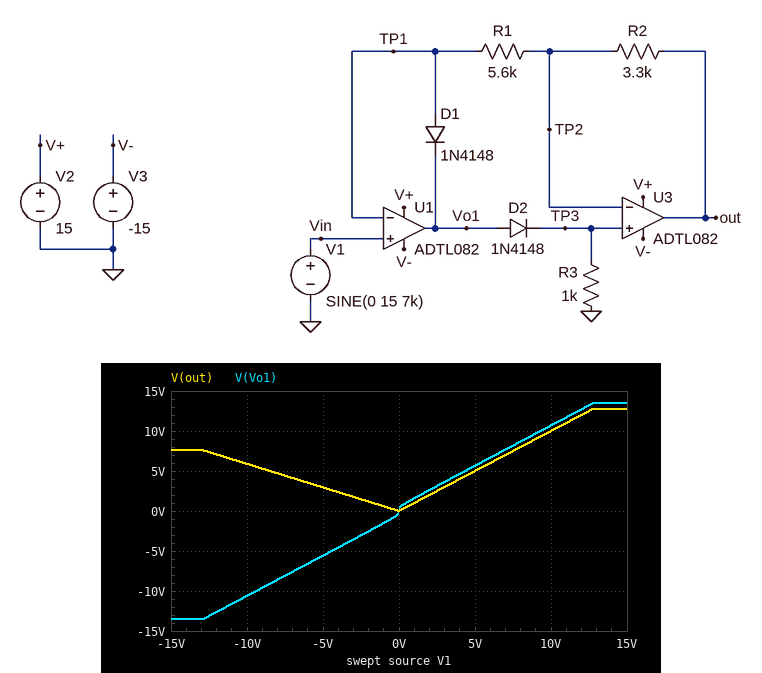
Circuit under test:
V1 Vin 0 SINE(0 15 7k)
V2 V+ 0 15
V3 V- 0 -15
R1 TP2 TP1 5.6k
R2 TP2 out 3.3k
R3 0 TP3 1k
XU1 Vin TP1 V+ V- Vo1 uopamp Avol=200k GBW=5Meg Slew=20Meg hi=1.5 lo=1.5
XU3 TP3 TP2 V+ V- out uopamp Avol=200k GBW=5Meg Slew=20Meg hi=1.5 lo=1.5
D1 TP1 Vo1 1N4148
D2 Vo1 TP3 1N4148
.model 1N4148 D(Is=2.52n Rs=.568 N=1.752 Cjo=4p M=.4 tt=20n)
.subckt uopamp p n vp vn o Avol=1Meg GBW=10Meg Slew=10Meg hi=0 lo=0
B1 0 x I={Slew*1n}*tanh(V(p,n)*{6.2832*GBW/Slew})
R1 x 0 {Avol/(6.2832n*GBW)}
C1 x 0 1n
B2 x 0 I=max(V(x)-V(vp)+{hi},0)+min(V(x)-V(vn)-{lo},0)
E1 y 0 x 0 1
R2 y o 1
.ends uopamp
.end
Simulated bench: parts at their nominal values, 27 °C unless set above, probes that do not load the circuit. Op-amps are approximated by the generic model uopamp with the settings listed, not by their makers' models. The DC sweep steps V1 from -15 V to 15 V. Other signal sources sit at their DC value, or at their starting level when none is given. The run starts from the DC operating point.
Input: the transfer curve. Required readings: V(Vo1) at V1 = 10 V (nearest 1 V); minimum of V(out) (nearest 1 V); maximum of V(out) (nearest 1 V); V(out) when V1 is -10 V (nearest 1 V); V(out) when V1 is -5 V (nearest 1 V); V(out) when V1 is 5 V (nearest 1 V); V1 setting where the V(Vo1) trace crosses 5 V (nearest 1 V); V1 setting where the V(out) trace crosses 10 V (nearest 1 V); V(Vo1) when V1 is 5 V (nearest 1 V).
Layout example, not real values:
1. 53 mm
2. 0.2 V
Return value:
1. 11 V
2. 0 V
3. 13 V
4. 6 V
5. 3 V
6. 5 V
7. 4 V
8. 10 V
9. 6 V
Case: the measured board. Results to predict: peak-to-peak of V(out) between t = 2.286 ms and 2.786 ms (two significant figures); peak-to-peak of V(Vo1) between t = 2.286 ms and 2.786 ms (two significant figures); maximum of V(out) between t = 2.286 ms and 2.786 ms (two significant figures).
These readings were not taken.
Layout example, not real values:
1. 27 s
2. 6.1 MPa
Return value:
1. 13 V
2. 27 V
3. 13 V
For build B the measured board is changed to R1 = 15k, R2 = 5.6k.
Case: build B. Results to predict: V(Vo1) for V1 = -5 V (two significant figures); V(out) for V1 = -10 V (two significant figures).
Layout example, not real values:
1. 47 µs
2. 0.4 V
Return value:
1. -5.5 V
2. 3.7 V
